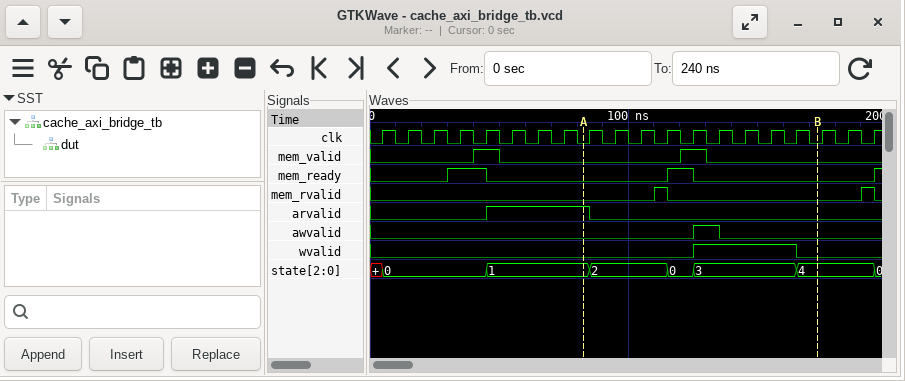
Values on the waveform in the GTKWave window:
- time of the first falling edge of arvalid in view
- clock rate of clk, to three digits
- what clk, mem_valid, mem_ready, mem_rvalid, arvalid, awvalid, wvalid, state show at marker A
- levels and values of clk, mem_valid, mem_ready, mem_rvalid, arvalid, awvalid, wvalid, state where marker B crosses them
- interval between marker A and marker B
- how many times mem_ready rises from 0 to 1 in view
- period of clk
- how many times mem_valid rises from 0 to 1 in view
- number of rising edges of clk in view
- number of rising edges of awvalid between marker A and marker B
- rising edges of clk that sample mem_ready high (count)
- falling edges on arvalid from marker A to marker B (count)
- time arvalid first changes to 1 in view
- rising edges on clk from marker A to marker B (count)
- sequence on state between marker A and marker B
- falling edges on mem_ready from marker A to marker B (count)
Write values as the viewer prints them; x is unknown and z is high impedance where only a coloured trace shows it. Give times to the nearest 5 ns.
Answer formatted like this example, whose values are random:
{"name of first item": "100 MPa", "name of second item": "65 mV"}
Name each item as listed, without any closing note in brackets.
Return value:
{"time of the first falling edge of arvalid in view": "85 ns", "clock rate of clk, to three digits": "100 MHz", "what clk, mem_valid, mem_ready, mem_rvalid, arvalid, awvalid, wvalid, state show at marker A": "clk=0, mem_valid=0, mem_ready=0, mem_rvalid=0, arvalid=1, awvalid=0, wvalid=0, state=1", "levels and values of clk, mem_valid, mem_ready, mem_rvalid, arvalid, awvalid, wvalid, state where marker B crosses them": "clk=0, mem_valid=0, mem_ready=0, mem_rvalid=0, arvalid=0, awvalid=0, wvalid=0, state=4", "interval between marker A and marker B": "90 ns", "how many times mem_ready rises from 0 to 1 in view": "3", "period of clk": "10 ns", "how many times mem_valid rises from 0 to 1 in view": "2", "number of rising edges of clk in view": "20", "number of rising edges of awvalid between marker A and marker B": "1", "rising edges of clk that sample mem_ready high": "3", "falling edges on arvalid from marker A to marker B": "1", "time arvalid first changes to 1 in view": "45 ns", "rising edges on clk from marker A to marker B": "9", "sequence on state between marker A and marker B": "1, 2, 0, 3, 4", "falling edges on mem_ready from marker A to marker B": "1"}
